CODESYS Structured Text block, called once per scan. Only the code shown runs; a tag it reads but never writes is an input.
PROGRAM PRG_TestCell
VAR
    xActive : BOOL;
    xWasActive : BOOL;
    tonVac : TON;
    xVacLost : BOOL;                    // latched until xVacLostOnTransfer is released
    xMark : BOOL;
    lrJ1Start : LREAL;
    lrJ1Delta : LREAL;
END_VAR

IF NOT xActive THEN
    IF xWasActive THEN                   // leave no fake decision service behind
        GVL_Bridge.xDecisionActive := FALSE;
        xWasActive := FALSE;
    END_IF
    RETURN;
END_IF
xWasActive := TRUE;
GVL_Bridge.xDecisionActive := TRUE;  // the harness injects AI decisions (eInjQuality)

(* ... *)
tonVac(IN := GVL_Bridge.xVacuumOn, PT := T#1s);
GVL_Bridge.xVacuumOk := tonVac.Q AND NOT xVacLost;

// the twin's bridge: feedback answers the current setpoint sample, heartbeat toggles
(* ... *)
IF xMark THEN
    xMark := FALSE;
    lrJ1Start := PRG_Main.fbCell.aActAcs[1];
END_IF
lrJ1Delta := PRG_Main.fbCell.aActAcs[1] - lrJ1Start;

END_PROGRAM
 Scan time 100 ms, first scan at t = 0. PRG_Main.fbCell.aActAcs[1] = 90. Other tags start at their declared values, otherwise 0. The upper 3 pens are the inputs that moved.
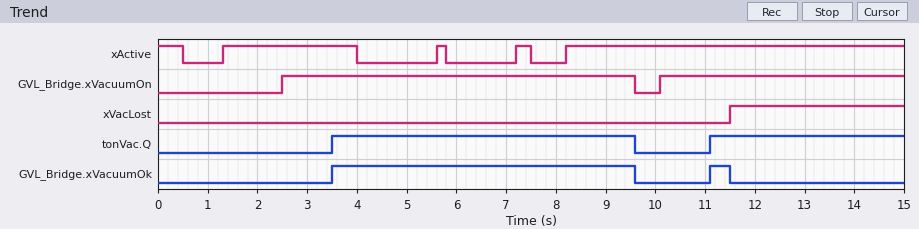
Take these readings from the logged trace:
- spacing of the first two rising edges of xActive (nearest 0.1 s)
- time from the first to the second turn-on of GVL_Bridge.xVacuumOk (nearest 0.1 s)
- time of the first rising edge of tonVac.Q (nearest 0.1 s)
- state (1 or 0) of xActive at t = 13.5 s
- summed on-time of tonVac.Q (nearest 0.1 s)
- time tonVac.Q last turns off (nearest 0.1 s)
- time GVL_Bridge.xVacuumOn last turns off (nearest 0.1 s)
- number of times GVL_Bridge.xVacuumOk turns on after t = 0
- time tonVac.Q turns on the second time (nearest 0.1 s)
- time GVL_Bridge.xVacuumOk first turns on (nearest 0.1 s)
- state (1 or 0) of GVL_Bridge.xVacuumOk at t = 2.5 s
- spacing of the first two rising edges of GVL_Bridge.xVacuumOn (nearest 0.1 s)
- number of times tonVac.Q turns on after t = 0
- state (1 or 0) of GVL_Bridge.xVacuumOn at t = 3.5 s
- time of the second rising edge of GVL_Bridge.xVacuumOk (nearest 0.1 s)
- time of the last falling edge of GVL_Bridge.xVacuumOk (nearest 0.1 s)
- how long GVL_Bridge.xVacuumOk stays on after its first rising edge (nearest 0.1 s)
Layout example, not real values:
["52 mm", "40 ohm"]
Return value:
["4.3 s", "7.6 s", "3.5 s", "1", "10.0 s", "9.6 s", "9.6 s", "2", "11.1 s", "3.5 s", "0", "7.6 s", "2", "1", "11.1 s", "11.5 s", "6.1 s"]
